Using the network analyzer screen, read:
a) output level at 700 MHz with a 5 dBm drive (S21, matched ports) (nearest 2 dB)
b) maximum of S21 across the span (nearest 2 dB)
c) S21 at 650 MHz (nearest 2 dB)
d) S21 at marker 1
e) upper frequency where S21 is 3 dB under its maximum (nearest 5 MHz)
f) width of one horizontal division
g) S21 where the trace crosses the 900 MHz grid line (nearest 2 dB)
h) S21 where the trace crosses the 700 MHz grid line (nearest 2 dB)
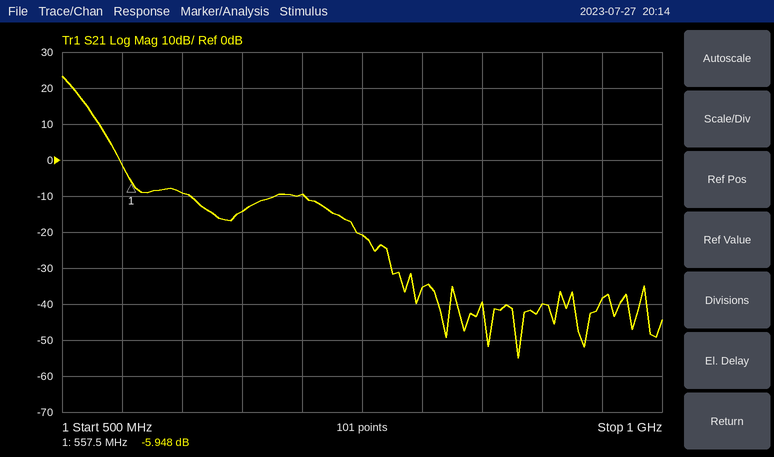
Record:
-4 dBm
24 dB
-14 dB
-5.948 dB
510 MHz
50 MHz
-40 dB
-10 dB
